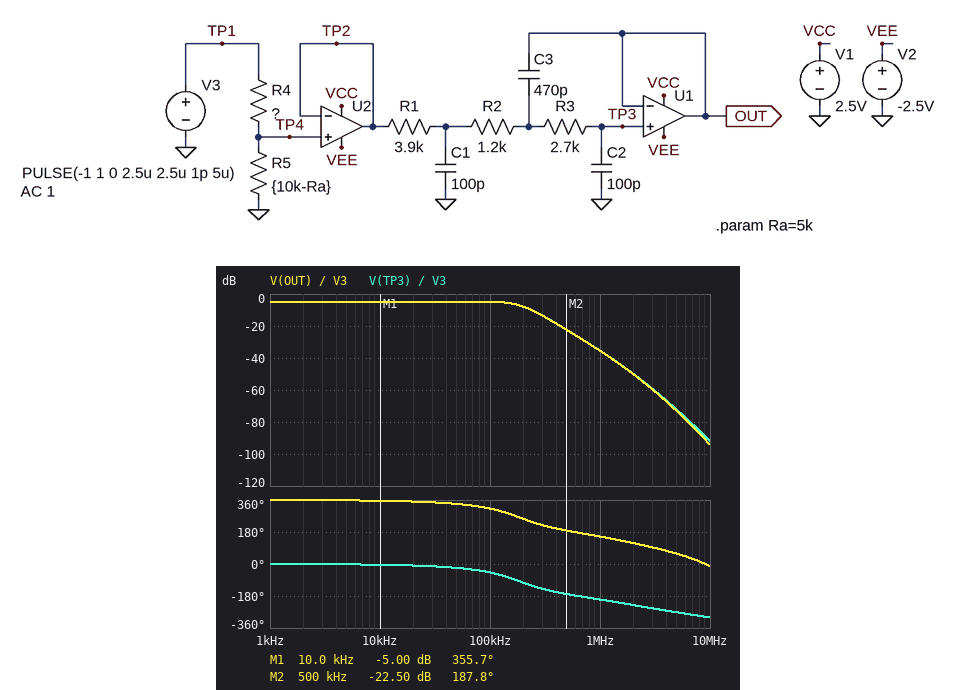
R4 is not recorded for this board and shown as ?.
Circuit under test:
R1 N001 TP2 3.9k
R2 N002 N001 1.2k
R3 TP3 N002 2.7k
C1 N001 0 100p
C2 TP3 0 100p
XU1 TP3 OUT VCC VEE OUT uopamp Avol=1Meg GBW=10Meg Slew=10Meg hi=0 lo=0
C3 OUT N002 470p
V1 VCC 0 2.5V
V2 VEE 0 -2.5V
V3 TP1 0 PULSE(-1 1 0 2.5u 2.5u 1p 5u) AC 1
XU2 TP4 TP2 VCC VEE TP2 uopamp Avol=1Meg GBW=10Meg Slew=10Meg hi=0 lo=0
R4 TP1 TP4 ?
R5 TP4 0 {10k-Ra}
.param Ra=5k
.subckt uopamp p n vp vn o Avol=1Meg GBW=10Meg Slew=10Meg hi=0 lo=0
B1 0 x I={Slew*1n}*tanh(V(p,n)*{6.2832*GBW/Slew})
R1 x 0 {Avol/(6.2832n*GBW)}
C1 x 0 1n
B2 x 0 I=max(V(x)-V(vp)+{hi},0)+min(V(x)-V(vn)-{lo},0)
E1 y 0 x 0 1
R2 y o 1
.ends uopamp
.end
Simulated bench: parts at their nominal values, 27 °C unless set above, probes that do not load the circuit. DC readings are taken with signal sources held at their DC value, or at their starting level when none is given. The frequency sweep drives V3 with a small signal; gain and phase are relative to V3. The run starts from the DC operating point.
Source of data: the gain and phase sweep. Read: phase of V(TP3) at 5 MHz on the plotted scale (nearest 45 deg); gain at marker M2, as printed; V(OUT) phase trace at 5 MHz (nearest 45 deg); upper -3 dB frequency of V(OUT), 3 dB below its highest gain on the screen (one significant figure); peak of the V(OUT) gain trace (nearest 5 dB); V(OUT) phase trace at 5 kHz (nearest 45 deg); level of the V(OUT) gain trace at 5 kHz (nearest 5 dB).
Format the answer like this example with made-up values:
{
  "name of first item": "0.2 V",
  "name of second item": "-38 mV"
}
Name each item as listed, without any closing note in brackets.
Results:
{
  "phase of V(TP3) at 5 MHz on the plotted scale": "-270 deg",
  "gain at marker M2, as printed": "-22.50 dB",
  "V(OUT) phase trace at 5 MHz": "45 deg",
  "upper -3 dB frequency of V(OUT), 3 dB below its highest gain on the screen": "200 kHz",
  "peak of the V(OUT) gain trace": "-5 dB",
  "V(OUT) phase trace at 5 kHz": "360 deg",
  "level of the V(OUT) gain trace at 5 kHz": "-5 dB"
}
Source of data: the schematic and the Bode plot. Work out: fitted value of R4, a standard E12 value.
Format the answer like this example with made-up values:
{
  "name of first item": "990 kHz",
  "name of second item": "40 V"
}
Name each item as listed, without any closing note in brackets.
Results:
{
  "fitted value of R4, a standard E12 value": "3.9 kΩ"
}
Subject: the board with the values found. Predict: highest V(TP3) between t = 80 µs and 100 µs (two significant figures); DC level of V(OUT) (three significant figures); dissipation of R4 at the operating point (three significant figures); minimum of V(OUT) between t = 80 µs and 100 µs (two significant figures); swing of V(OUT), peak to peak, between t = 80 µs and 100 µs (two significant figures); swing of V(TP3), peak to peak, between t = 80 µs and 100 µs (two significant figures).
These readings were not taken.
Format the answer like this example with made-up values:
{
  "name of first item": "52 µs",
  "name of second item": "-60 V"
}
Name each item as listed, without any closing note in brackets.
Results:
{
  "highest V(TP3) between t = 80 µs and 100 µs": "330 mV",
  "DC level of V(OUT)": "-562 mV",
  "dissipation of R4 at the operating point": "49.2 µW",
  "minimum of V(OUT) between t = 80 µs and 100 µs": "-330 mV",
  "swing of V(OUT), peak to peak, between t = 80 µs and 100 µs": "650 mV",
  "swing of V(TP3), peak to peak, between t = 80 µs and 100 µs": "650 mV"
}
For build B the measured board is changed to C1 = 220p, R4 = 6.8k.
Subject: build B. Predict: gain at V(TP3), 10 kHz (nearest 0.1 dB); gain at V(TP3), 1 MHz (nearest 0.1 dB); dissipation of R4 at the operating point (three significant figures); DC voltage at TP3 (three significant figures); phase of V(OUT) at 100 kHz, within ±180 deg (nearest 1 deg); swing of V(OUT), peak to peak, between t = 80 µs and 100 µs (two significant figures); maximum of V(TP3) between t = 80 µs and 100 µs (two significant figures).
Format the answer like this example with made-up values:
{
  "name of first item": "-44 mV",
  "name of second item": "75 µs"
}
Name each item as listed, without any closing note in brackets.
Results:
{
  "gain at V(TP3), 10 kHz": "-7.5 dB",
  "gain at V(TP3), 1 MHz": "-40.8 dB",
  "dissipation of R4 at the operating point": "48.8 µW",
  "DC voltage at TP3": "-424 mV",
  "phase of V(OUT) at 100 kHz, within ±180 deg": "-60 deg",
  "swing of V(OUT), peak to peak, between t = 80 µs and 100 µs": "360 mV",
  "maximum of V(TP3) between t = 80 µs and 100 µs": "180 mV"
}
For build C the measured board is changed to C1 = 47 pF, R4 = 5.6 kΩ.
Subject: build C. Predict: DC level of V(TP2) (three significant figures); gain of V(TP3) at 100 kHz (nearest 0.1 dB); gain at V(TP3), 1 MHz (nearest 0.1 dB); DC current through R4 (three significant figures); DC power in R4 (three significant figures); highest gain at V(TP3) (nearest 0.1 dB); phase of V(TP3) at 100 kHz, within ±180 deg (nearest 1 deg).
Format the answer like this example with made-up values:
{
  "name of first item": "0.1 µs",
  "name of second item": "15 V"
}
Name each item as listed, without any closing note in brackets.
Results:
{
  "DC level of V(TP2)": "-472 mV",
  "gain of V(TP3) at 100 kHz": "-5.8 dB",
  "gain at V(TP3), 1 MHz": "-35.8 dB",
  "DC current through R4": "94.3 µA",
  "DC power in R4": "49.8 µW",
  "highest gain at V(TP3)": "-5.7 dB",
  "phase of V(TP3) at 100 kHz, within ±180 deg": "-41 deg"
}
